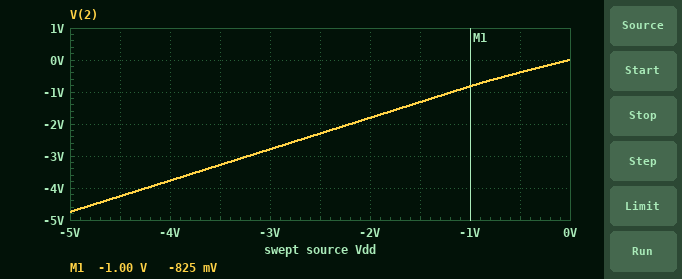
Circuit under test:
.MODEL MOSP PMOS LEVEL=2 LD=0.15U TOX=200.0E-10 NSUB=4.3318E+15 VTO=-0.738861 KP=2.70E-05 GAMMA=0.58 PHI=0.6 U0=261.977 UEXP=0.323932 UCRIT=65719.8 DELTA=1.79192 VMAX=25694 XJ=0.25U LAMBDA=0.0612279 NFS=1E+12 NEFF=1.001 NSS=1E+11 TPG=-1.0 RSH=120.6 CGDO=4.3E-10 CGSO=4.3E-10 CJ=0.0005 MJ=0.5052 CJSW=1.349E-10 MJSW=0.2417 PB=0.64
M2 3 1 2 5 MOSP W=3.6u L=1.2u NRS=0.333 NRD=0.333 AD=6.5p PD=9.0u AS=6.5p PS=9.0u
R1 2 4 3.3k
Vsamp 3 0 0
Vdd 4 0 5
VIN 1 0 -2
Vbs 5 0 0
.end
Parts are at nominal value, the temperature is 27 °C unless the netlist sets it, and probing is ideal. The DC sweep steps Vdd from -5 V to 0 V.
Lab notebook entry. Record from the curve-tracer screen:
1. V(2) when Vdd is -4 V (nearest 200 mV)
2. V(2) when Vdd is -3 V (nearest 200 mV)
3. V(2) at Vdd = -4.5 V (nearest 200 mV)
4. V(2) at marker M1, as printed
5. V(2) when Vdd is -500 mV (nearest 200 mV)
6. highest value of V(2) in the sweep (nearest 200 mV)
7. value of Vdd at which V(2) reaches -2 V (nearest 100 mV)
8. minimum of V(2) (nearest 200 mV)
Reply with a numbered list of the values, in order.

1. -3.8 V
2. -2.8 V
3. -4.2 V
4. -825 mV
5. -400 mV
6. 0 V
7. -2.2 V
8. -4.8 V
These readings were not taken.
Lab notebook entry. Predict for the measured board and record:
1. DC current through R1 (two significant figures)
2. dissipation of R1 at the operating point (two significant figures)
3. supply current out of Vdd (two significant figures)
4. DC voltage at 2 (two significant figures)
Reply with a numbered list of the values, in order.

1. 1.3 mA
2. 5.6 mW
3. 1.3 mA
4. 710 mV
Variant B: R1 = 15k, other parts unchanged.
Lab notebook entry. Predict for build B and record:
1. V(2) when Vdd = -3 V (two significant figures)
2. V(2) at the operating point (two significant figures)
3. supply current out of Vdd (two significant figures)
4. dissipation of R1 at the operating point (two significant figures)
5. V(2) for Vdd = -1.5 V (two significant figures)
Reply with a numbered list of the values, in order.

1. -2.1 V
2. 630 mV
3. 290 µA
4. 1.3 mW
5. -720 mV
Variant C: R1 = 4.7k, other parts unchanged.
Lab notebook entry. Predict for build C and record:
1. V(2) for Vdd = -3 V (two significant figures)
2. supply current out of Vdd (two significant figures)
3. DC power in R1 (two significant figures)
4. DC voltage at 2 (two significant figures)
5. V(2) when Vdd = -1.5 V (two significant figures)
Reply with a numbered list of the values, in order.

1. -2.7 V
2. 920 µA
3. 4.0 mW
4. 690 mV
5. -1.2 V
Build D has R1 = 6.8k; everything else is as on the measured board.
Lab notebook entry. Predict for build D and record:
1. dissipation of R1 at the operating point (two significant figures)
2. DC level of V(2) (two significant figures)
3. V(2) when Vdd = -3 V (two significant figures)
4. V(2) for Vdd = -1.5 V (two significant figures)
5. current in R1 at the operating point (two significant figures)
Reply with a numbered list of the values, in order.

1. 2.8 mW
2. 670 mV
3. -2.6 V
4. -1.1 V
5. 640 µA
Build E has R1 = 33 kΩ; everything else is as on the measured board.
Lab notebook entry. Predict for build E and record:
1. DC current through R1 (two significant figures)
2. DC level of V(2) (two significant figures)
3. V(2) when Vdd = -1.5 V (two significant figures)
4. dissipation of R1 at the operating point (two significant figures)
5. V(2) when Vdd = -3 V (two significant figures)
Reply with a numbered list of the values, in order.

1. 130 µA
2. 590 mV
3. -390 mV
4. 590 µW
5. -1.2 V
